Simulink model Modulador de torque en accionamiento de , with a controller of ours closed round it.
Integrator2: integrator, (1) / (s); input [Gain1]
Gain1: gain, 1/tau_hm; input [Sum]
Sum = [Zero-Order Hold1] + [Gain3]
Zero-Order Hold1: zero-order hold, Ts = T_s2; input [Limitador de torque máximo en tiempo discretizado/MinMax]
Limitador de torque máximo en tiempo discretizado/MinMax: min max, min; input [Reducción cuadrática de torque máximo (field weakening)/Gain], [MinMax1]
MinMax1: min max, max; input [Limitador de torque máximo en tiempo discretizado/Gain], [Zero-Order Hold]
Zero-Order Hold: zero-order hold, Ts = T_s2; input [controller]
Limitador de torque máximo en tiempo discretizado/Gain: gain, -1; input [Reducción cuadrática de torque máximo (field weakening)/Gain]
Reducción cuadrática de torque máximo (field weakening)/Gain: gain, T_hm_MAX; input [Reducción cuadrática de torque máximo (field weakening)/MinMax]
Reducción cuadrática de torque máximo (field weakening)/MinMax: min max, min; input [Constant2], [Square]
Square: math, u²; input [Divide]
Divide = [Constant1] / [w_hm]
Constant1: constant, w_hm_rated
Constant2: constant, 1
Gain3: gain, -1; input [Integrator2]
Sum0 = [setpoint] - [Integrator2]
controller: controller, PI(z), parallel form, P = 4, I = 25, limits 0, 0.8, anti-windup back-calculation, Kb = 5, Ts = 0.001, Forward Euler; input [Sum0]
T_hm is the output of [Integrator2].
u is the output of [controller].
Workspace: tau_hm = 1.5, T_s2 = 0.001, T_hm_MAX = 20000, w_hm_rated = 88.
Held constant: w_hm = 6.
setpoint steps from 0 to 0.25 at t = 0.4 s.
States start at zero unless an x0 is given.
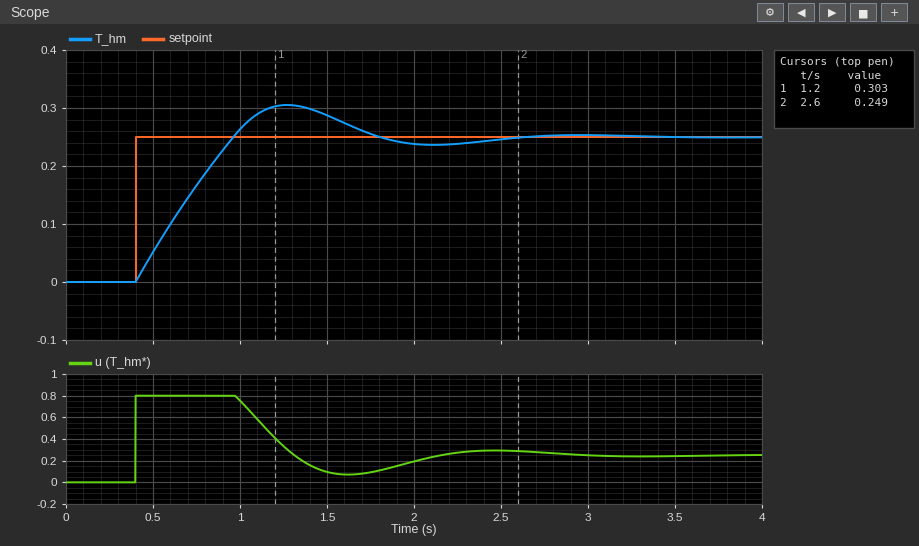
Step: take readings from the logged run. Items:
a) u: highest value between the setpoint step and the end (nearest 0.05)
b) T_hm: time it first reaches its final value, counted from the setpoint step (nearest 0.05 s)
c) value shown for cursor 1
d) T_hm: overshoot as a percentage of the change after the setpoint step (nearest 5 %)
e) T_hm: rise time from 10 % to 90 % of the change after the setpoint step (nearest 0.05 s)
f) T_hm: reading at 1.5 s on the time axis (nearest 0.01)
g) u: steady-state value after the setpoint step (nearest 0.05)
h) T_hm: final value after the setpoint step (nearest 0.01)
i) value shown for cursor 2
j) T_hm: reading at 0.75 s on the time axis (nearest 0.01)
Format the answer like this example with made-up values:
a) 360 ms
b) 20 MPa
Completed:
a) 0.80
b) 0.55 s
c) 0.303
d) 20 %
e) 0.45 s
f) 0.29
g) 0.25
h) 0.25
i) 0.249
j) 0.17
